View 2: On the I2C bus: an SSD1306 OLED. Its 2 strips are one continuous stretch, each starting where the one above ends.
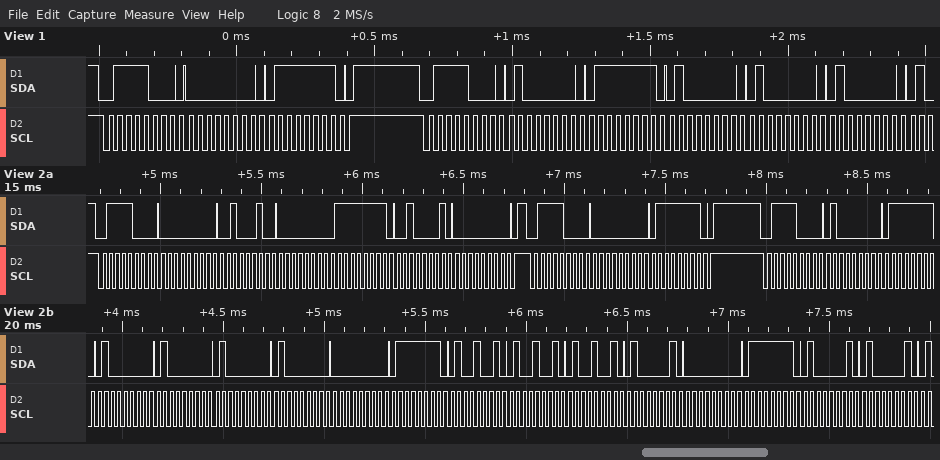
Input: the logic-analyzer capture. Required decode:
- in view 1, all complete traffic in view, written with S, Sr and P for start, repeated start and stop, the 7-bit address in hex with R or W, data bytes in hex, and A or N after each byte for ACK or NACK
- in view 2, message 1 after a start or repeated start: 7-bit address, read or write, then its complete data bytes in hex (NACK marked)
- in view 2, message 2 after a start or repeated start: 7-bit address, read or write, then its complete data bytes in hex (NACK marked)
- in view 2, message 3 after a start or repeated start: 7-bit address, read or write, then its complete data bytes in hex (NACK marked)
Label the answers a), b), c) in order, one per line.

a) S 3CW A 00 A 7F A P S 3CW A 40 A 7F A 40 A 40 A 40 A
b) 0x3C write: 00 22 00 FF 21 00
c) 0x3C write: 00 7F
d) 0x3C write: 40 7F 40 40 40 40 00 7F 49 49 49 41 00 7F 41 41
